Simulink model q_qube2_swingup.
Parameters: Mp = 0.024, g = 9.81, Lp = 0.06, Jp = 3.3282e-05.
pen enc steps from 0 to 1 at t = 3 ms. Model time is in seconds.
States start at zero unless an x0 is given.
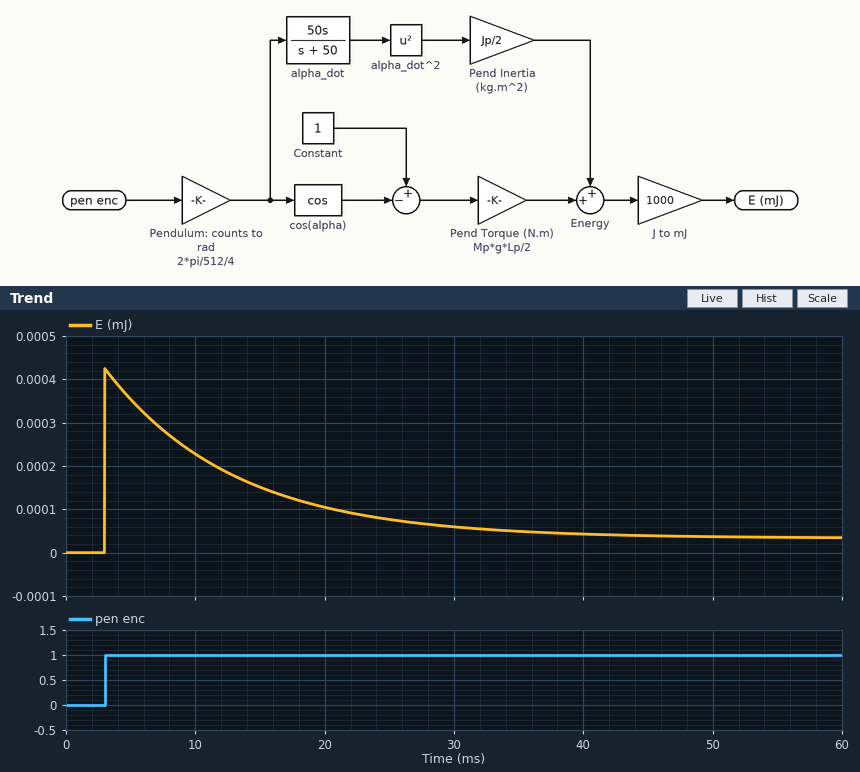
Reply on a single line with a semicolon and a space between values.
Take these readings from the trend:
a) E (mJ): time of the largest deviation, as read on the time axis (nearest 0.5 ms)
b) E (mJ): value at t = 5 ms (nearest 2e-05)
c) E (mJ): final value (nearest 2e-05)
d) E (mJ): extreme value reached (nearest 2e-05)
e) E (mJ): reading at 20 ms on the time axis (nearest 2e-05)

3.0 ms; 0.00036; 0.00004; 0.00042; 0.00010
